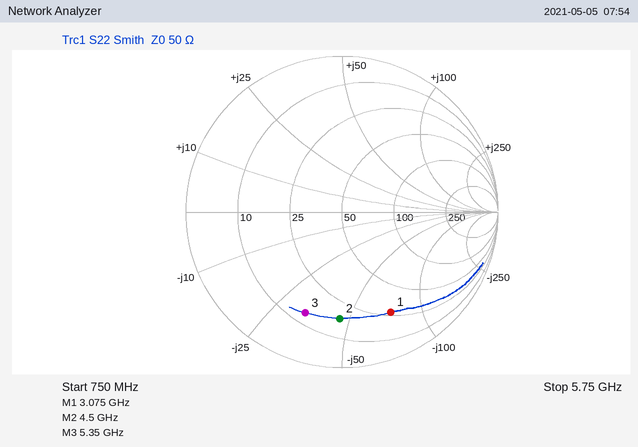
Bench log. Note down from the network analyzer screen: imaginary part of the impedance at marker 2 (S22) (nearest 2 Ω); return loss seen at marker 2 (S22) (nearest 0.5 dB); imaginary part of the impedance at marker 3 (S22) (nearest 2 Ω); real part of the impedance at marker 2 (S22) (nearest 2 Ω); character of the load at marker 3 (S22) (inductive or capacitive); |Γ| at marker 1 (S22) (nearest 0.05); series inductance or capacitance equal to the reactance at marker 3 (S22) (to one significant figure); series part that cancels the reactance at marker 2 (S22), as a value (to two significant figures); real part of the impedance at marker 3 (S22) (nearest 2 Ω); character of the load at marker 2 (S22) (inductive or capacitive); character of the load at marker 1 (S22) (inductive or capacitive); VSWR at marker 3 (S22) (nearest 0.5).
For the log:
-46 Ω
3.5 dB
-34 Ω
18 Ω
capacitive
0.70
900 fF
1.6 nH
14 Ω
capacitive
capacitive
5.5
